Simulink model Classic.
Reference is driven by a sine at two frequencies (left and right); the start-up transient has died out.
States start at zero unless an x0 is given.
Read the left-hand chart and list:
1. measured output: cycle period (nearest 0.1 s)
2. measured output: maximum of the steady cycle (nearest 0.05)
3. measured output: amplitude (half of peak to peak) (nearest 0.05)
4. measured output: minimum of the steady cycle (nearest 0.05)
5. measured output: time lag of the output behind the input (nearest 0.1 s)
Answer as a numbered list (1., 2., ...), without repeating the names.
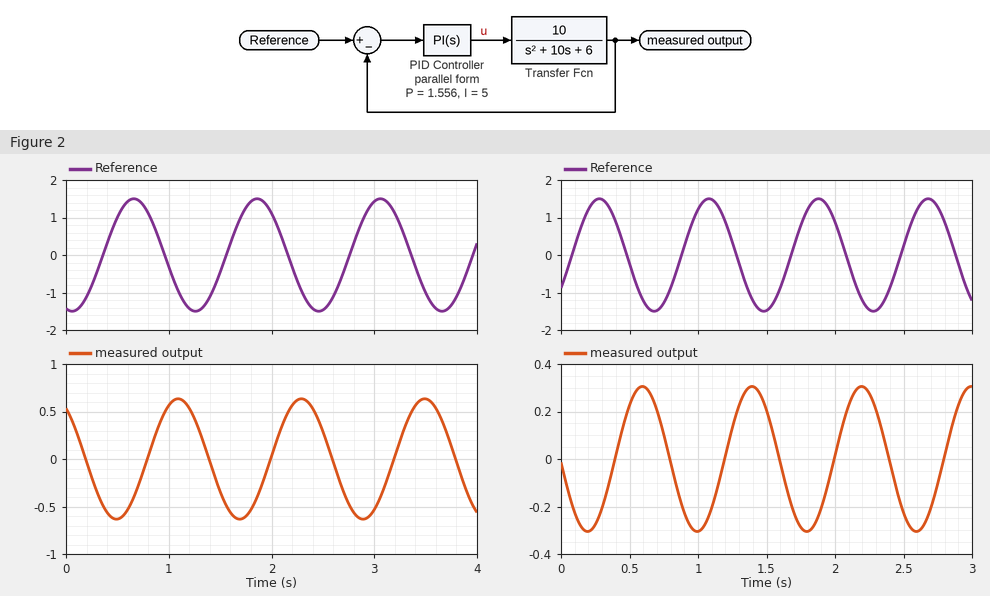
1. 1.2 s
2. 0.65
3. 0.65
4. -0.65
5. 0.4 s
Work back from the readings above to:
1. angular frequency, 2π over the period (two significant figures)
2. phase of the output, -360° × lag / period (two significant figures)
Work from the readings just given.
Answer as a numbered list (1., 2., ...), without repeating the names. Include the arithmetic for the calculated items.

1. 2π / 1.2 = 5.2 rad/s
2. -360 × 0.4 / 1.2 = -120°
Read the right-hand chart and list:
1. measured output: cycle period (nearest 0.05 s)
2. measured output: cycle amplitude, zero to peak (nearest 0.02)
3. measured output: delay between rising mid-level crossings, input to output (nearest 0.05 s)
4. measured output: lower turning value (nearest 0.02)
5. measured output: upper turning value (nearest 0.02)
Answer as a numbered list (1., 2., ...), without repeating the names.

1. 0.80 s
2. 0.30
3. 0.30 s
4. -0.30
5. 0.30
